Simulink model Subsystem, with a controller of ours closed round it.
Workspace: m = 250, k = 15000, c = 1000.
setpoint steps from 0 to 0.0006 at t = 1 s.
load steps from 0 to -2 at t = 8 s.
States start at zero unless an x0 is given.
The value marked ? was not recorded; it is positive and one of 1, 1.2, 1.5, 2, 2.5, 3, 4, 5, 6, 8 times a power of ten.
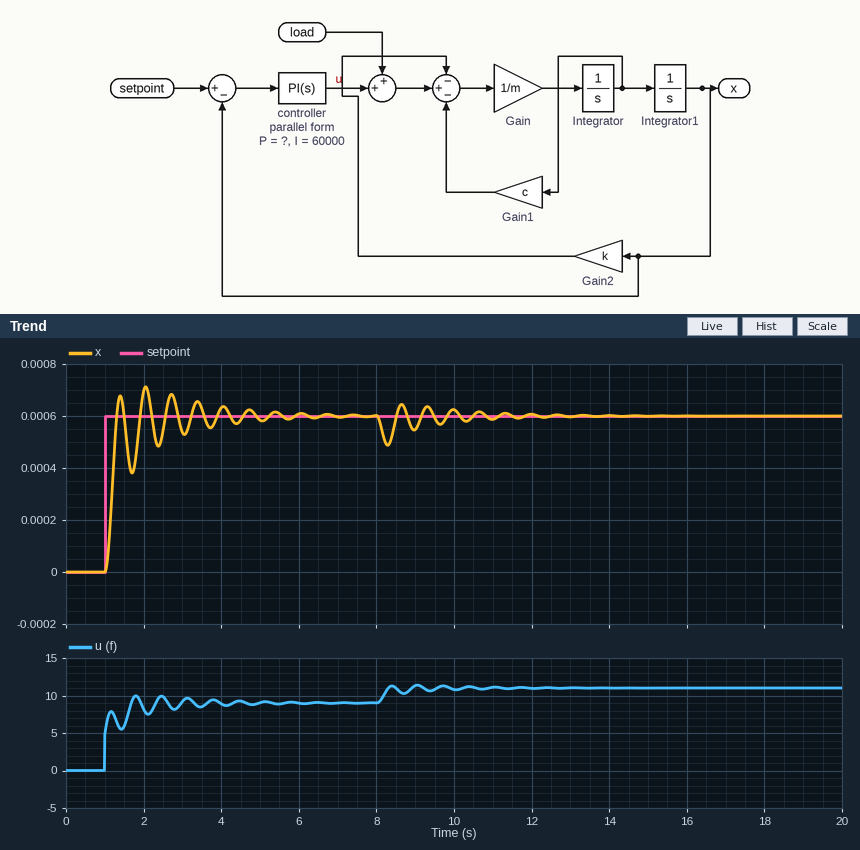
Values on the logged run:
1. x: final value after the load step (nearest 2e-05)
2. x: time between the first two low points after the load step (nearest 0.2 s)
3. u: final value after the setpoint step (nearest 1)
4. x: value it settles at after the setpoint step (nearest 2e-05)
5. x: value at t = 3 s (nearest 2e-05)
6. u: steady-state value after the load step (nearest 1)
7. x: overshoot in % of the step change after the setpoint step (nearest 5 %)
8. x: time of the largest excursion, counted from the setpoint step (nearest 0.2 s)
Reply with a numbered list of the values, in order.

1. 0.00060
2. 0.6 s
3. 9
4. 0.00060
5. 0.00054
6. 11
7. 20 %
8. 1.0 s
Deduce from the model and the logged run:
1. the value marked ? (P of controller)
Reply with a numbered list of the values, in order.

1. 8000
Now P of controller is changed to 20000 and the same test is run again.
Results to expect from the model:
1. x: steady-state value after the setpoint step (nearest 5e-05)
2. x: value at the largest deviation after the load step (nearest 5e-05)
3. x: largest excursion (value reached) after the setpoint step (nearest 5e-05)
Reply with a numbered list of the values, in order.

1. 0.00060
2. 0.00050
3. 0.00070
